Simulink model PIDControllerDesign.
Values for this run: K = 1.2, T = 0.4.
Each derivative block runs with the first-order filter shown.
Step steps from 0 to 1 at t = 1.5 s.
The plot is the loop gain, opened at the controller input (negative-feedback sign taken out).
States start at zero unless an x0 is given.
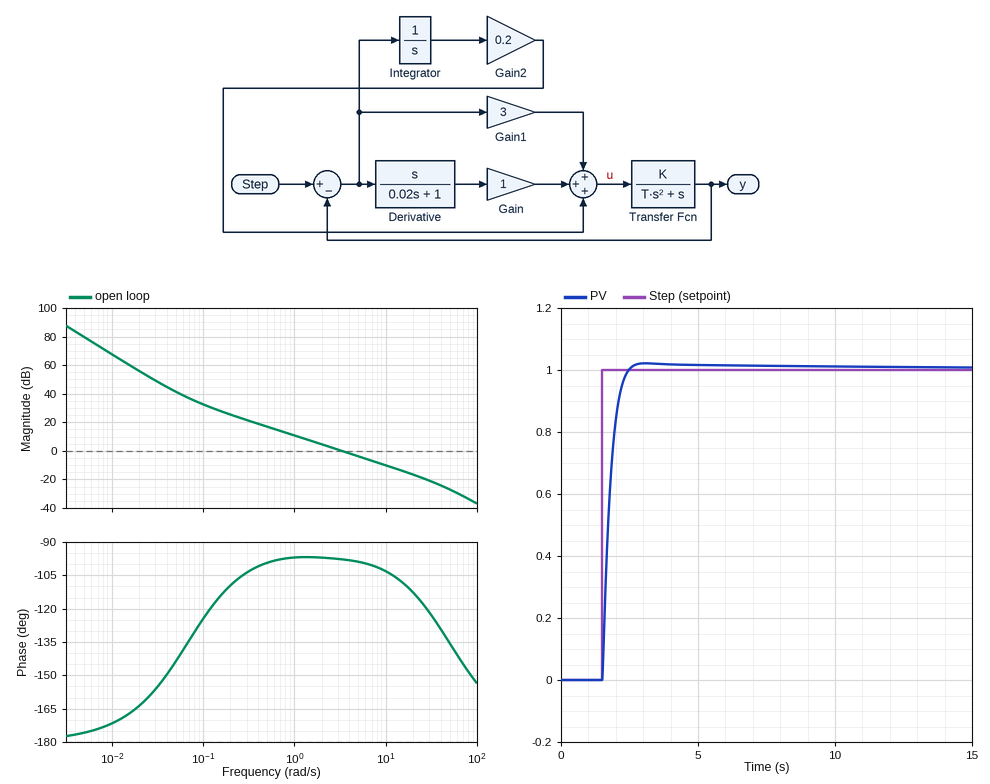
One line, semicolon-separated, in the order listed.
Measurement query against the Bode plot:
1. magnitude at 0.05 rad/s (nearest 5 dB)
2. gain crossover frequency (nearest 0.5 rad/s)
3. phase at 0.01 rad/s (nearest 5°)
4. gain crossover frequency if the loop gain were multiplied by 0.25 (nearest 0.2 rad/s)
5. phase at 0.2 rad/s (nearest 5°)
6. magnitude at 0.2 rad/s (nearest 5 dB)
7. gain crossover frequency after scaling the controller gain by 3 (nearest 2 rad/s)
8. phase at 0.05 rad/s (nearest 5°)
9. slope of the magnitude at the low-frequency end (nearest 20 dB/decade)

40 dB; 3.5 rad/s; -170°; 0.8 rad/s; -110°; 25 dB; 10 rad/s; -145°; -40 dB/decade
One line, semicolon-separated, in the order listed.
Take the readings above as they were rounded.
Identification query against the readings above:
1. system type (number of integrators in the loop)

2
